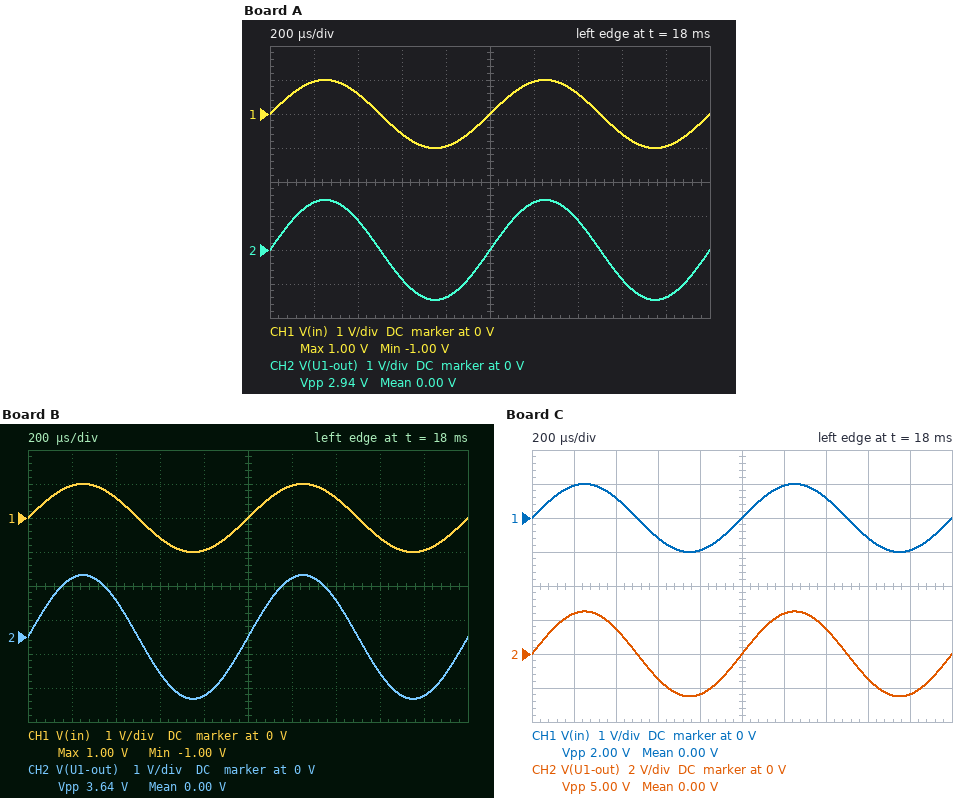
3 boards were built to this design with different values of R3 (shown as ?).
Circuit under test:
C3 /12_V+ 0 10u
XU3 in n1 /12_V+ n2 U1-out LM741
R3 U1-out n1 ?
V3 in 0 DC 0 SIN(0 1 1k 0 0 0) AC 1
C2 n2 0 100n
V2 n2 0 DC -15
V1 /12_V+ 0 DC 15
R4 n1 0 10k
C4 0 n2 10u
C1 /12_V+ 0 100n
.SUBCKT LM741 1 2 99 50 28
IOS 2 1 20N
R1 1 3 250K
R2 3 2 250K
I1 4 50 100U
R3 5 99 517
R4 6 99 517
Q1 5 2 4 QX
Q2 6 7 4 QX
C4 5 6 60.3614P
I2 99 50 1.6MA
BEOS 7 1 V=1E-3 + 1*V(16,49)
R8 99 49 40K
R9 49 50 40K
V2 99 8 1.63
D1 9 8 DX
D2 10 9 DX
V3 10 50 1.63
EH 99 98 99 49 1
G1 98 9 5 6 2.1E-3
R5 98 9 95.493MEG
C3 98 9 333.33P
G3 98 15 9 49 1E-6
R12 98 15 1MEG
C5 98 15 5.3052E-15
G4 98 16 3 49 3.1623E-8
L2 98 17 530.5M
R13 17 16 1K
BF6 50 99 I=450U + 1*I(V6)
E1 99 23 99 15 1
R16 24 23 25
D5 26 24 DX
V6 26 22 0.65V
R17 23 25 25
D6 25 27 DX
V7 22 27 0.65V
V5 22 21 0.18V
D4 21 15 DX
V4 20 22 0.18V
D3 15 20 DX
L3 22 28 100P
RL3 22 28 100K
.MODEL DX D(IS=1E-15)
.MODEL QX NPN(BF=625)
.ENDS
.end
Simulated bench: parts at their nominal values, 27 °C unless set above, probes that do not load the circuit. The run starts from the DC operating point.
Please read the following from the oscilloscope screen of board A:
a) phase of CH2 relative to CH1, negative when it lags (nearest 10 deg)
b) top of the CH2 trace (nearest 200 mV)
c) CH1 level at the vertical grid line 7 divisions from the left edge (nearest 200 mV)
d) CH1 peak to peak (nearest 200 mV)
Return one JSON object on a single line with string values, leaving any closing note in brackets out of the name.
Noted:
{"phase of CH2 relative to CH1, negative when it lags": "0 deg", "top of the CH2 trace": "1.4 V", "CH1 level at the vertical grid line 7 divisions from the left edge": "600 mV", "CH1 peak to peak": "2.0 V"}
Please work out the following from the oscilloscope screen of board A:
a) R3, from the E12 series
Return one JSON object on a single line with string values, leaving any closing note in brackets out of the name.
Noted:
{"R3, from the E12 series": "4.7 kΩ"}
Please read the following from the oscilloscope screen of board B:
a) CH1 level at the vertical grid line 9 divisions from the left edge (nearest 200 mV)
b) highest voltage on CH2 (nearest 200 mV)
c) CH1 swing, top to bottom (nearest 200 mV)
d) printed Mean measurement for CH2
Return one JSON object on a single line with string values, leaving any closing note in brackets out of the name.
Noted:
{"CH1 level at the vertical grid line 9 divisions from the left edge": "-1.0 V", "highest voltage on CH2": "1.8 V", "CH1 swing, top to bottom": "2.0 V", "printed Mean measurement for CH2": "0.00 V"}
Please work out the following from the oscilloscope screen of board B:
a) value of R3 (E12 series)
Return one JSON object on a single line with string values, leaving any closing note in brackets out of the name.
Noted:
{"value of R3": "8.2 kΩ"}
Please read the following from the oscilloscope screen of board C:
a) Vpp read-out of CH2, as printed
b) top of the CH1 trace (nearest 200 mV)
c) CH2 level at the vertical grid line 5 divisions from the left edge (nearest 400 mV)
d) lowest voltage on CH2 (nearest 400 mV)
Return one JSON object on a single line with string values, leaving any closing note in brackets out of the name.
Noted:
{"Vpp read-out of CH2, as printed": "5.00 V", "top of the CH1 trace": "1.0 V", "CH2 level at the vertical grid line 5 divisions from the left edge": "0 V", "lowest voltage on CH2": "-2.4 V"}
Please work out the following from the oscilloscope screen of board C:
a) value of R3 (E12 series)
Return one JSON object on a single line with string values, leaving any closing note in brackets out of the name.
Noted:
{"value of R3": "15 kΩ"}
